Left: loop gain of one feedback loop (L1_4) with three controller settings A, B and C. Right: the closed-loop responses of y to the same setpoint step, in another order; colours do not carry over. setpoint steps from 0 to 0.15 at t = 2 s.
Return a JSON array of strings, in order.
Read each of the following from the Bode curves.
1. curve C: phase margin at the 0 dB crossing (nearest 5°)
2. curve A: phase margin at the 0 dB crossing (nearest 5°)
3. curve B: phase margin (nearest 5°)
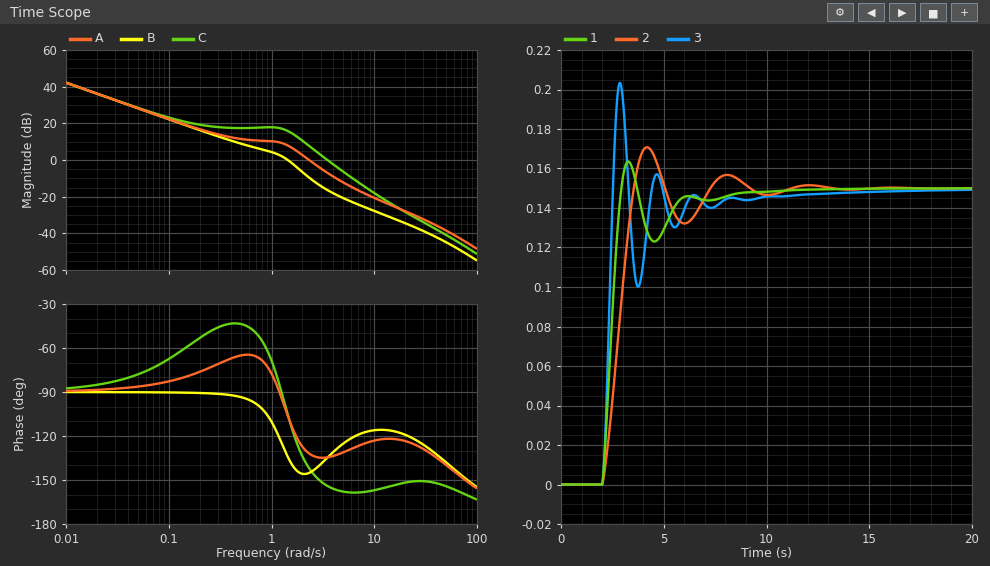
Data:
["25°", "50°", "45°"]
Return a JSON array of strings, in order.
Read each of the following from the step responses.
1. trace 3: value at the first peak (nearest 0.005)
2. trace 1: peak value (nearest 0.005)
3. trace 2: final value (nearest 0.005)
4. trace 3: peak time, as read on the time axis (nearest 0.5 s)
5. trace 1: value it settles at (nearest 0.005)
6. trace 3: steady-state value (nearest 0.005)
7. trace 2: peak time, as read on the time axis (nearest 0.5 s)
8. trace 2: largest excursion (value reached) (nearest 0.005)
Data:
["0.205", "0.165", "0.150", "3.0 s", "0.150", "0.150", "4.0 s", "0.170"]
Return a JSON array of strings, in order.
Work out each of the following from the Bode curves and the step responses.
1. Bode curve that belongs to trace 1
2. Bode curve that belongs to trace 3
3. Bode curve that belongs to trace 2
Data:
["A", "C", "B"]
